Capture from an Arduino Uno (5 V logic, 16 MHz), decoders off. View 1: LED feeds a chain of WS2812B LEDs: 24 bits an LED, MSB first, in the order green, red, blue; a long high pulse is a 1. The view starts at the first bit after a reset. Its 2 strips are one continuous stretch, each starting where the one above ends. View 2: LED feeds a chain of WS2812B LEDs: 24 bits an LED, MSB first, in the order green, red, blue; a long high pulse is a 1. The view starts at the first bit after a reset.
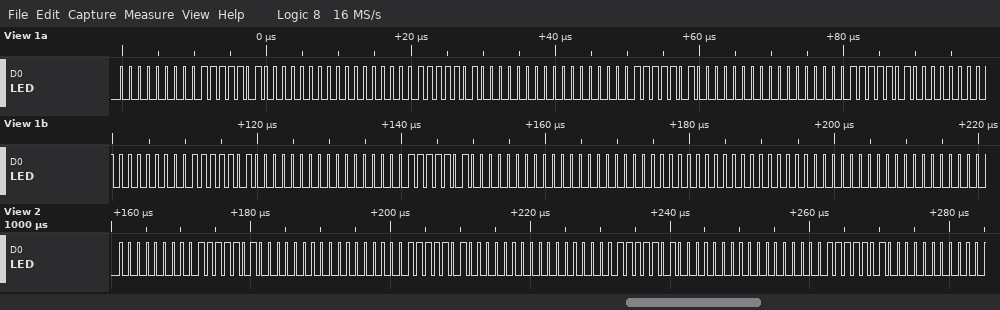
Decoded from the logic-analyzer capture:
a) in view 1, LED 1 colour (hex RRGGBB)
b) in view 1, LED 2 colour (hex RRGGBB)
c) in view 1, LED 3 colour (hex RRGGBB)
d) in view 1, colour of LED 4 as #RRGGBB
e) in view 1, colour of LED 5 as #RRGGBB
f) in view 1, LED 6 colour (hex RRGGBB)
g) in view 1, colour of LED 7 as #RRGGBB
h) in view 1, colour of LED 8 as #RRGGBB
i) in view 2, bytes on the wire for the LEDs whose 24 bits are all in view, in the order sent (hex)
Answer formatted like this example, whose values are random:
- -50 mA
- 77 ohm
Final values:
- #7D0000
- #7D0000
- #7D0000
- #7D0000
- #7D0000
- #7D0000
- #000000
- #000000
- 00 7D 00 00 7D 00 00 7D 00 00 7D 00
